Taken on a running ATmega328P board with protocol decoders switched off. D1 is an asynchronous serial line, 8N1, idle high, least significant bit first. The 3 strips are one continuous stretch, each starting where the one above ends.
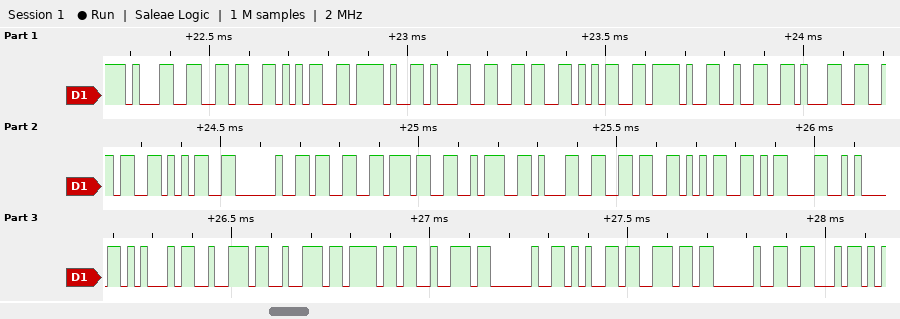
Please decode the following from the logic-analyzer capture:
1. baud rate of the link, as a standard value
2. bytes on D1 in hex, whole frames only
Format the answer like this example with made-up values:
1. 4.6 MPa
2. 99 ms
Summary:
1. 57600 baud
2. 31 36 35 2F 31 36 35 2F 32 31 36 35 20 33 37 3A 31 36 35 0D 0A 45 72 72 6F 72 20 65 6E 20 46
